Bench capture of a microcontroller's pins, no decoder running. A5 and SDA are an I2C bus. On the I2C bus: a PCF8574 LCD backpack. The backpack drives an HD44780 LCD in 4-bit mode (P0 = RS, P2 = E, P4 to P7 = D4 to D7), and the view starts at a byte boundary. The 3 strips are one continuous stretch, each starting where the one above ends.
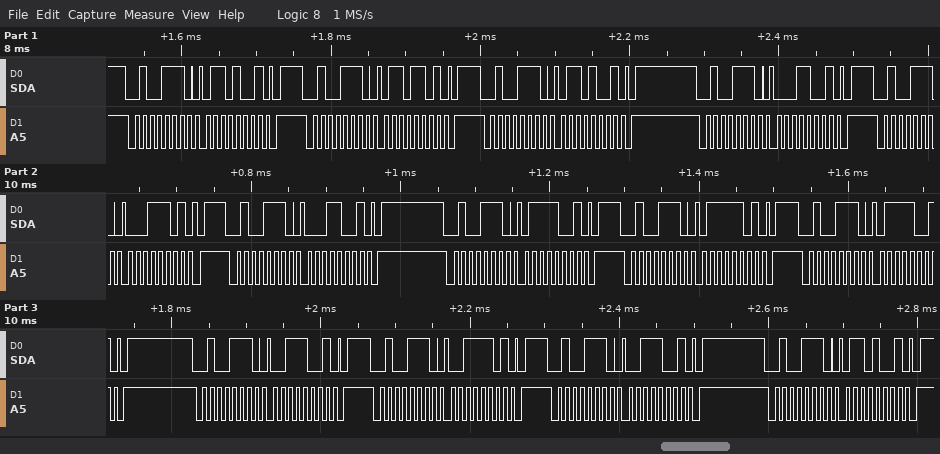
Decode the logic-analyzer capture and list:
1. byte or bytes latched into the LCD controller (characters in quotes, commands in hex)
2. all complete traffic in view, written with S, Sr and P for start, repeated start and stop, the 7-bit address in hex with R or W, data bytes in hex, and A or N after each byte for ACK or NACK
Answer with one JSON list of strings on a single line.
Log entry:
["'a' 's'", "S 27W A 69 A P S 27W A 6D A P S 27W A 69 A P S 27W A 19 A P S 27W A 1D A P S 27W A 19 A P S 27W A 79 A P S 27W A 7D A P S 27W A 79 A P S 27W A 39 A P S 27W A 3D A P S 27W A 39 A P S 27W A 69 A P"]
